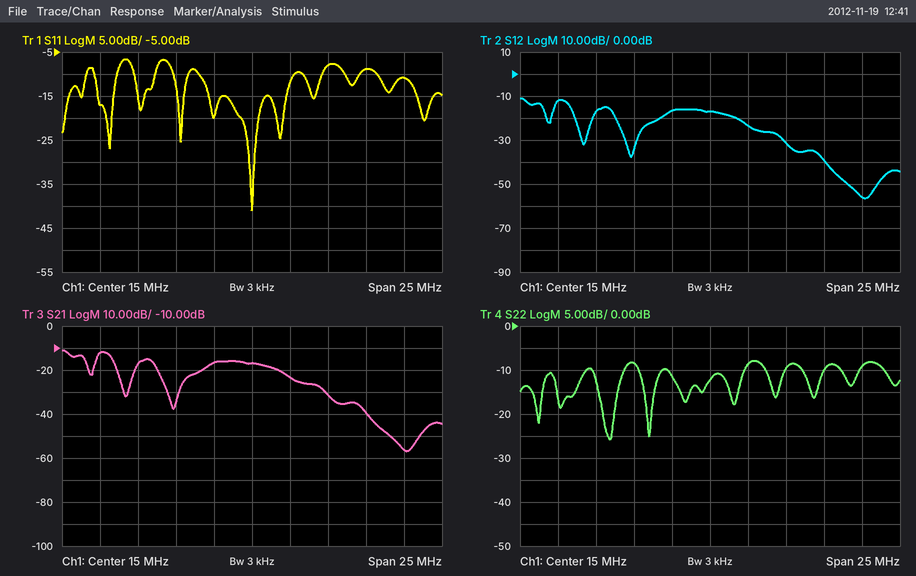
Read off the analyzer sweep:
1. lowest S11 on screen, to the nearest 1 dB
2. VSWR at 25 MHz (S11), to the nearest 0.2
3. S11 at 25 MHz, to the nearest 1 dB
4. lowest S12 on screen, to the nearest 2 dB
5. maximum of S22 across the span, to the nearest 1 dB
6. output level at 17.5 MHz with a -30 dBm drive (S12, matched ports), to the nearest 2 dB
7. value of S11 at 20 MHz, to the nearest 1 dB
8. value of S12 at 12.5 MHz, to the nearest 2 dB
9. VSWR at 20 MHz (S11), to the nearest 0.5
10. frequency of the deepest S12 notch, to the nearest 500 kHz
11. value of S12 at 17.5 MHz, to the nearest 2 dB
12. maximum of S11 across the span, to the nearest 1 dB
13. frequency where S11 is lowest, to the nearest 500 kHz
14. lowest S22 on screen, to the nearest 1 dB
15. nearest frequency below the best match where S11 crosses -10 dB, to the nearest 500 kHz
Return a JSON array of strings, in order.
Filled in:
["-41 dB", "1.8", "-11 dB", "-56 dB", "-8 dB", "-54 dBm", "-8 dB", "-16 dB", "2.5", "25.0 MHz", "-24 dB", "-7 dB", "15.0 MHz", "-26 dB", "11.5 MHz"]
